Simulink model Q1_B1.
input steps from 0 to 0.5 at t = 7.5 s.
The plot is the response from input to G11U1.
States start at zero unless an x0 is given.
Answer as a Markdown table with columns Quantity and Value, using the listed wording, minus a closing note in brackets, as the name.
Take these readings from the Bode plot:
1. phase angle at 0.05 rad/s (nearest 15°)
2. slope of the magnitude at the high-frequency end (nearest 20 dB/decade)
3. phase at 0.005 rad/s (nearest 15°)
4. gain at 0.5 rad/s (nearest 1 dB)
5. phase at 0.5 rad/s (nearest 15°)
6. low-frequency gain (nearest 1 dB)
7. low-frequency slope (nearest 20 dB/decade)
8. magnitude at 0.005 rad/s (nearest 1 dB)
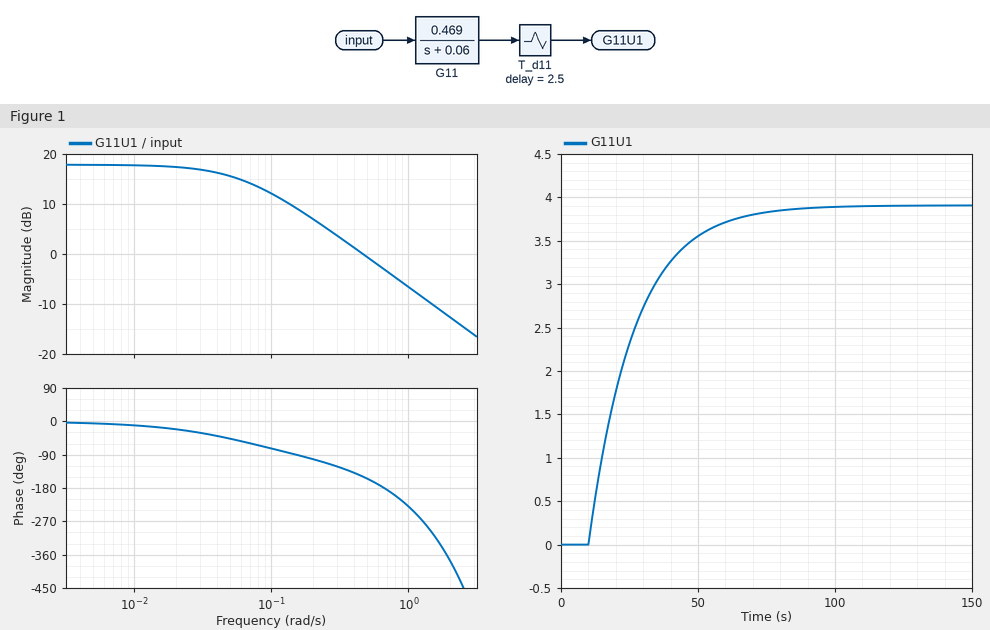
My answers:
| Quantity | Value |
|---|---|
| phase angle at 0.05 rad/s | -45° |
| slope of the magnitude at the high-frequency end | -20 dB/decade |
| phase at 0.005 rad/s | 0° |
| gain at 0.5 rad/s | -1 dB |
| phase at 0.5 rad/s | -150° |
| low-frequency gain | 18 dB |
| low-frequency slope | 0 dB/decade |
| magnitude at 0.005 rad/s | 18 dB |
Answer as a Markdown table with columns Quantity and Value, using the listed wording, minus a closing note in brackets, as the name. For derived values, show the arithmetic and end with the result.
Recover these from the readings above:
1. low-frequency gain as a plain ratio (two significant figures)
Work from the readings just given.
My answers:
| Quantity | Value |
|---|---|
| low-frequency gain as a plain ratio | 10^(18 / 20) = 7.9 |
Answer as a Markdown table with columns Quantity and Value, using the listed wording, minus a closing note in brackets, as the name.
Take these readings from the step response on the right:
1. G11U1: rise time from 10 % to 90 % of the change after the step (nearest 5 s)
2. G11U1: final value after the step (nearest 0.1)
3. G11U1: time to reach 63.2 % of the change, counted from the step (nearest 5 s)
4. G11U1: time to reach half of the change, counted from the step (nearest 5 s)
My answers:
| Quantity | Value |
|---|---|
| G11U1: rise time from 10 % to 90 % of the change after the step | 35 s |
| G11U1: final value after the step | 3.9 |
| G11U1: time to reach 63.2 % of the change, counted from the step | 20 s |
| G11U1: time to reach half of the change, counted from the step | 15 s |
